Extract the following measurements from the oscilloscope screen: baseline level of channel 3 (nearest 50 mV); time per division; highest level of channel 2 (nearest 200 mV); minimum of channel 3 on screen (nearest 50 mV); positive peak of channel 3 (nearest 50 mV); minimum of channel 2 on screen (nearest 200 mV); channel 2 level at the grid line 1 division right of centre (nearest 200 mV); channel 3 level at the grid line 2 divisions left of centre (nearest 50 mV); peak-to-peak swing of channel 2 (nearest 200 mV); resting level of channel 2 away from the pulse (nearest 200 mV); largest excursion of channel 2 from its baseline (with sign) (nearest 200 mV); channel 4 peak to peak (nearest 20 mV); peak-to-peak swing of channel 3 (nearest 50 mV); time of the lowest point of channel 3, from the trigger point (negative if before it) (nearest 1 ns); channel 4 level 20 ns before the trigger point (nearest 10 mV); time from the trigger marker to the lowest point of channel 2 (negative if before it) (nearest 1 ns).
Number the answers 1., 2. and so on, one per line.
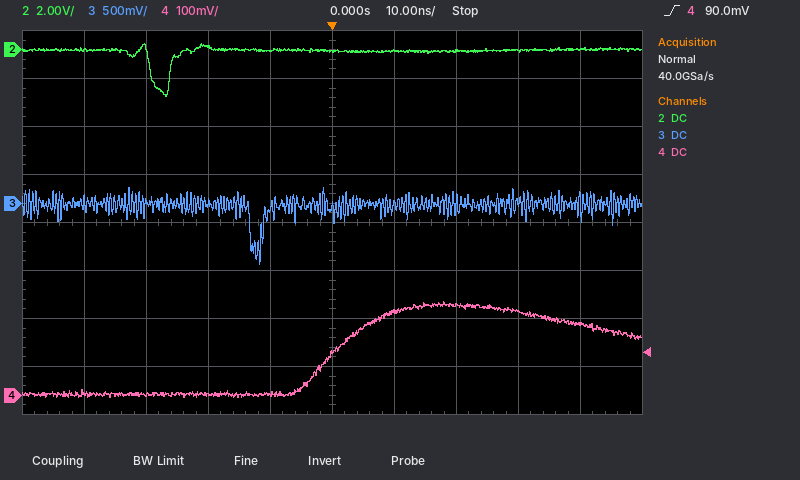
1. 0 mV
2. 10 ns
3. 200 mV
4. -650 mV
5. 150 mV
6. -2.0 V
7. 0.0 V
8. 0 mV
9. 2.2 V
10. 0.0 V
11. -2.0 V
12. 200 mV
13. 800 mV
14. -12 ns
15. 0 mV
16. -27 ns
